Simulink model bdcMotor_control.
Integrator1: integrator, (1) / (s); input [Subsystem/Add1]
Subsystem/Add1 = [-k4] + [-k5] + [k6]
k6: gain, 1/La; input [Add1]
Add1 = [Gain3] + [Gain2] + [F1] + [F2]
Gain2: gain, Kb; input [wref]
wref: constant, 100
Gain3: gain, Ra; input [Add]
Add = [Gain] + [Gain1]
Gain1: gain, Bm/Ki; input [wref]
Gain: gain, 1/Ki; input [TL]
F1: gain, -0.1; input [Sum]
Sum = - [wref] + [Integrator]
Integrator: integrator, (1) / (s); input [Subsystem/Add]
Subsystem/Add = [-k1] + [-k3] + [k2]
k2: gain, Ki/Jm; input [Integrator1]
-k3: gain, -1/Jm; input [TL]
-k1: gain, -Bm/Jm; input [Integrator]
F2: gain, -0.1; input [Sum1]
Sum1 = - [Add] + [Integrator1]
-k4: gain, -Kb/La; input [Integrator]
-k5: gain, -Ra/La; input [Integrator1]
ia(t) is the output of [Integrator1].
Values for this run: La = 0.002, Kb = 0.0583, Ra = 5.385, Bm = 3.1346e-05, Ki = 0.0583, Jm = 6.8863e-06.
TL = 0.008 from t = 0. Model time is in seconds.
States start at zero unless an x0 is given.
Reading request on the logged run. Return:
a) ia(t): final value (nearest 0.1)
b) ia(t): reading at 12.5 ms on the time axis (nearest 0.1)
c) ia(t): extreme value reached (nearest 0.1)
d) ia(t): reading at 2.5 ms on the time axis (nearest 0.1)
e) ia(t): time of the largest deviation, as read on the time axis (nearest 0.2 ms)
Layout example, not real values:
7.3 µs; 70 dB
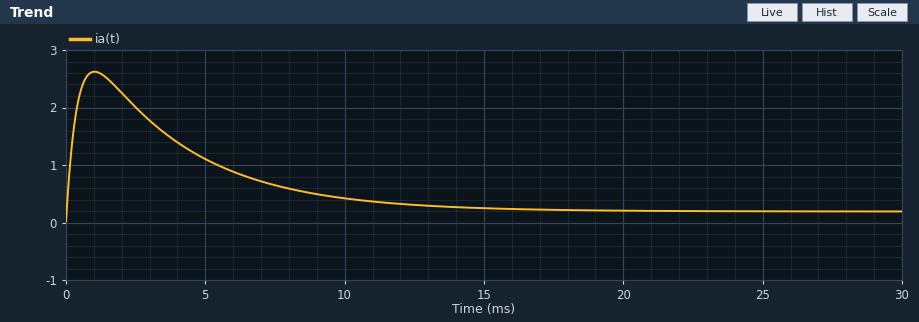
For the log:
0.2; 0.3; 2.6; 2.0; 1.0 ms
